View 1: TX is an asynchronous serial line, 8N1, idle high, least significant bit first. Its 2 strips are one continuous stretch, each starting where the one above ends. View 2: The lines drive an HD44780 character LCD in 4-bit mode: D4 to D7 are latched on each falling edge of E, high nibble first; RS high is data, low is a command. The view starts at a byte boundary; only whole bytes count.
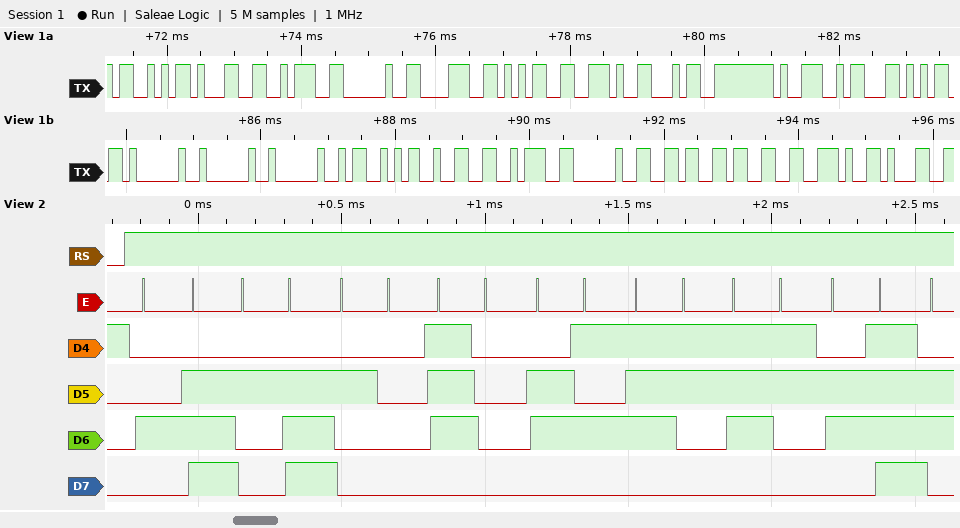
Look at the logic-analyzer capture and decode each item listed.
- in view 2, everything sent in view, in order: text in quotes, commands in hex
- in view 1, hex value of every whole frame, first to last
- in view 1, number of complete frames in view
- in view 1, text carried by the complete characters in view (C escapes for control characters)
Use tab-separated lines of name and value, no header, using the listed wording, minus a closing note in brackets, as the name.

in view 2, everything sent in view, in order: text in quotes, commands in hex	"N. pesso"
in view 1, hex value of every whole frame, first to last	53 31 3A 20 38 35 2E 34 39 63 6D 20 20 20 53 32 3A 20 36 33 2E 31
in view 1, number of complete frames in view	22
in view 1, text carried by the complete characters in view	"S1: 85.49cm   S2: 63.1"
